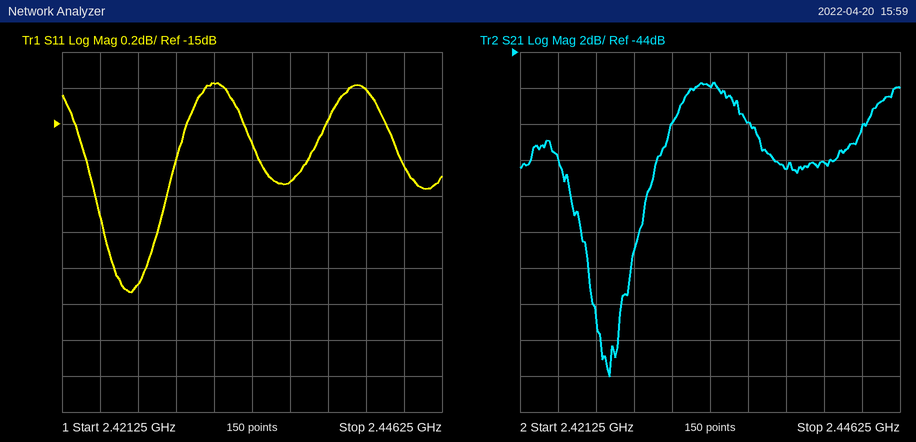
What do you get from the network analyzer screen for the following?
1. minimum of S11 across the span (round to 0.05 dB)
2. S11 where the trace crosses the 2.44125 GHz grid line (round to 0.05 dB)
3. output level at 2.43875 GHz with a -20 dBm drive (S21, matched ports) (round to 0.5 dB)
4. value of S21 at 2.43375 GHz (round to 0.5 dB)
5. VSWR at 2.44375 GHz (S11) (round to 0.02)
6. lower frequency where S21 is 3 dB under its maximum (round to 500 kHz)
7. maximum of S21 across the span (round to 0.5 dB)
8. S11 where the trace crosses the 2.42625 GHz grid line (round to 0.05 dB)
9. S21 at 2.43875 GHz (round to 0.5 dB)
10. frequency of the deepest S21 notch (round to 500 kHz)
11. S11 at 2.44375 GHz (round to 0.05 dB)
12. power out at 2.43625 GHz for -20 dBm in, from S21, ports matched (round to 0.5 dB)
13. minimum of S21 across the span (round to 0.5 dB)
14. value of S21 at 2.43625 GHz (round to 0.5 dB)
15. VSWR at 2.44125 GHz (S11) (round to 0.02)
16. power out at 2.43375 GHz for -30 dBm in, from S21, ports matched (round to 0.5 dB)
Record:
-15.95 dB
-14.80 dB
-70.5 dBm
-46.0 dB
1.42
2.4310 GHz
-45.5 dB
-15.90 dB
-50.5 dB
2.4270 GHz
-15.25 dB
-68.0 dBm
-62.0 dB
-48.0 dB
1.44
-76.0 dBm
